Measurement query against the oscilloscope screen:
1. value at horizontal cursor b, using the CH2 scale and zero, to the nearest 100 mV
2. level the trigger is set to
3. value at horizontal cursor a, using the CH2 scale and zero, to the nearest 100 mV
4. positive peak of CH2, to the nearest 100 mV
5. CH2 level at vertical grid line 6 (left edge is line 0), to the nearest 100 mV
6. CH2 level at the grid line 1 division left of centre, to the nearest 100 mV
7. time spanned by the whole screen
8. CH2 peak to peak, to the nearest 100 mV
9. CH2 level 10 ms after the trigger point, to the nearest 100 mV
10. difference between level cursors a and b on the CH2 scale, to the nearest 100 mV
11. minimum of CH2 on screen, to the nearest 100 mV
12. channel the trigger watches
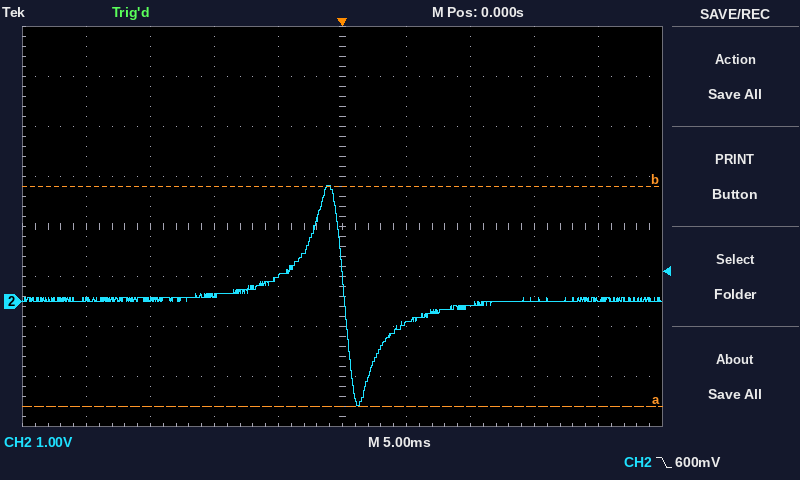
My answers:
2.3 V
600 mV
-2.1 V
2.3 V
-400 mV
500 mV
50 ms
4.4 V
-100 mV
4.4 V
-2.1 V
CH2
